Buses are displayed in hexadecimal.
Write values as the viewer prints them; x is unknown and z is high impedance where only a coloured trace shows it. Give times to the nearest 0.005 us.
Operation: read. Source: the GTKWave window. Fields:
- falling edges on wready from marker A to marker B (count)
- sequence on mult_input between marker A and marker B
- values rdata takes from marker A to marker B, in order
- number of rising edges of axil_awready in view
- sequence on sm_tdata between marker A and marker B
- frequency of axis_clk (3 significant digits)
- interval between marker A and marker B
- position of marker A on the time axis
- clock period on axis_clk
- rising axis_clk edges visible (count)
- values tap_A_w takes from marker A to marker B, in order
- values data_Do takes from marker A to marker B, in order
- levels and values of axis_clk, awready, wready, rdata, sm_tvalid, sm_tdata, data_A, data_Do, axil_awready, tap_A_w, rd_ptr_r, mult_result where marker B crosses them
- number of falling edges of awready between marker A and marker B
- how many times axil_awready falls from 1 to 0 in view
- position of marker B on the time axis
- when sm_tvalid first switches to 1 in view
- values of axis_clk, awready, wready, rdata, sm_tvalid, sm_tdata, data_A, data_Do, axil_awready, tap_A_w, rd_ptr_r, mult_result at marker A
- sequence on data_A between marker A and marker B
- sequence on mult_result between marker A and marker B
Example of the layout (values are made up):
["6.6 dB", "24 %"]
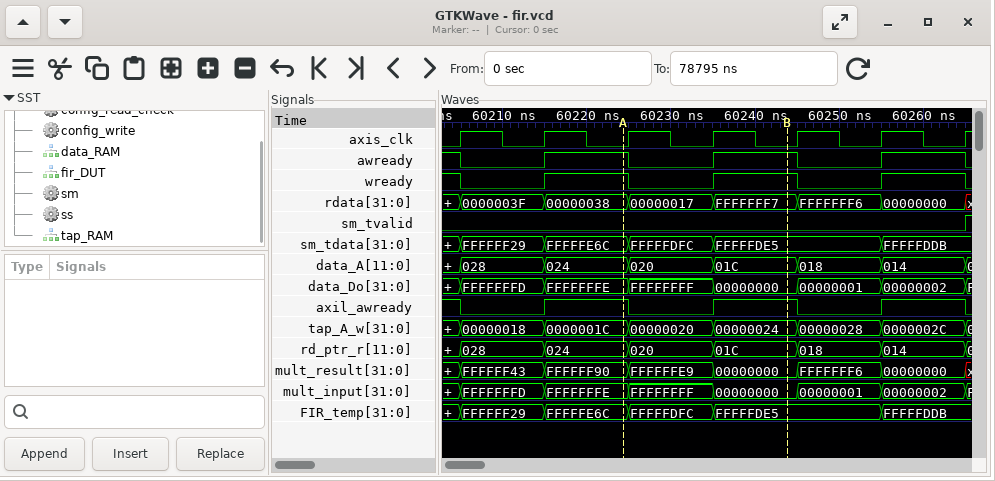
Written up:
["1", "FFFFFFFE, FFFFFFFF, 00000000", "00000038, 00000017, FFFFFFF7", "3", "FFFFFE6C, FFFFFDFC, FFFFFDE5", "100 MHz", "0.02 us", "60.225 us", "0.01 us", "7", "0000001C, 00000020, 00000024", "FFFFFFFE, FFFFFFFF, 00000000", "axis_clk=0, awready=1, wready=1, rdata=FFFFFFF7, sm_tvalid=0, sm_tdata=FFFFFDE5, data_A=01C, data_Do=00000000, axil_awready=1, tap_A_w=00000024, rd_ptr_r=01C, mult_result=00000000", "1", "4", "60.245 us", "60.265 us", "axis_clk=0, awready=1, wready=1, rdata=00000038, sm_tvalid=0, sm_tdata=FFFFFE6C, data_A=024, data_Do=FFFFFFFE, axil_awready=1, tap_A_w=0000001C, rd_ptr_r=024, mult_result=FFFFFF90", "024, 020, 01C", "FFFFFF90, FFFFFFE9, 00000000"]
